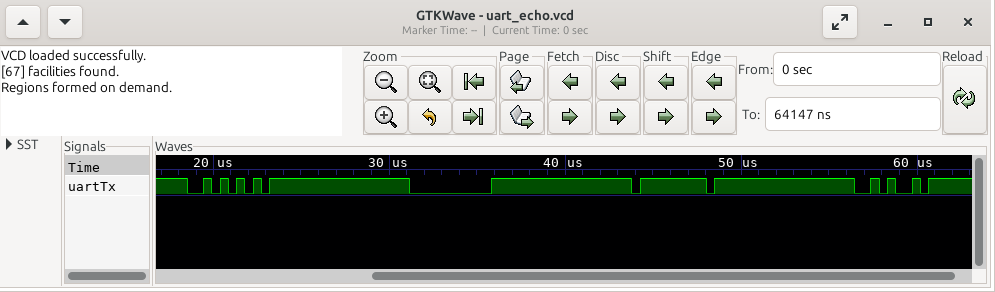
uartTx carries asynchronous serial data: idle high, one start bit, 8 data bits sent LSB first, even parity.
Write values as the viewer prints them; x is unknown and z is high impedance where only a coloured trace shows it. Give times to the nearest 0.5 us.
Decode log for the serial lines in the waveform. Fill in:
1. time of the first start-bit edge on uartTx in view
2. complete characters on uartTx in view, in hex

18.5 us
AA, 00, FF, 4A
